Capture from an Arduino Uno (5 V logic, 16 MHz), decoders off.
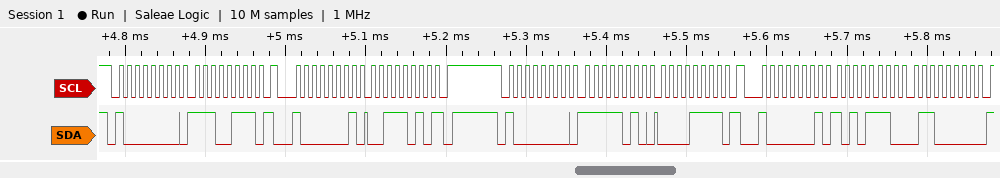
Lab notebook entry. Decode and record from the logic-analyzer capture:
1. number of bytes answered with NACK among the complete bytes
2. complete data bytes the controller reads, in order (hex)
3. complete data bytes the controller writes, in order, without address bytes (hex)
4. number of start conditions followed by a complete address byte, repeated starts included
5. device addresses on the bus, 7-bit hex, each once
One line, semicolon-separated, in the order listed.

1; 3A AE 60; E7 FA 0F; 4; 0x40
